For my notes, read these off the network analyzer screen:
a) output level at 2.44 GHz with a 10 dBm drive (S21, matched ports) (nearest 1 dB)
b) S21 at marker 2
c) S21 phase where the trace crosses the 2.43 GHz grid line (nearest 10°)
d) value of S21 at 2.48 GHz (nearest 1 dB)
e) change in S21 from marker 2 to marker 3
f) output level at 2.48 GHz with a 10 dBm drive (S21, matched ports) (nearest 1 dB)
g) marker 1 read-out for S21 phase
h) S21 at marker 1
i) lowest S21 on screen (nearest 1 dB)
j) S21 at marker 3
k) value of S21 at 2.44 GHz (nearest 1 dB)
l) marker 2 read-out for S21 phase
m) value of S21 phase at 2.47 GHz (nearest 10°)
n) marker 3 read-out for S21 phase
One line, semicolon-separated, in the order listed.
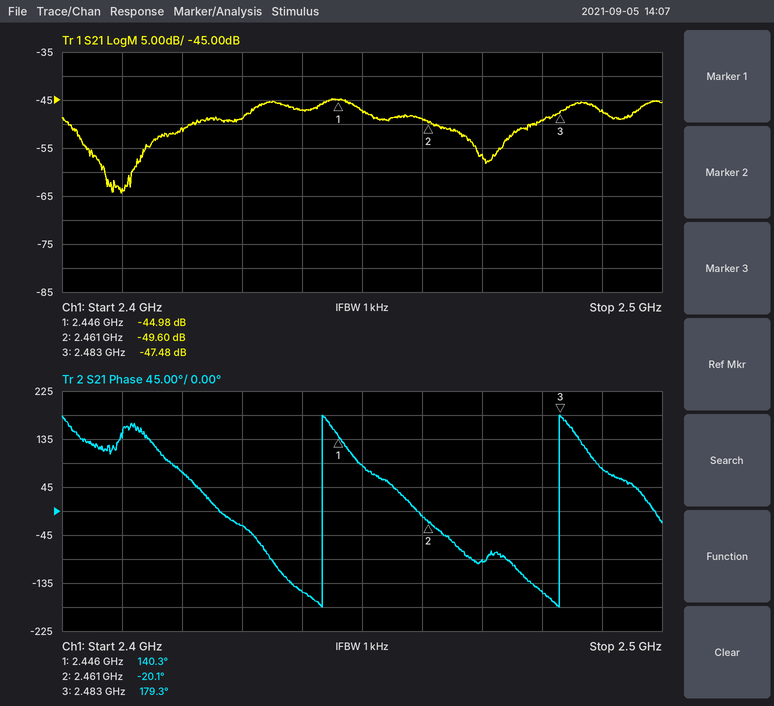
-37 dBm; -49.60 dB; -30°; -49 dB; 2.12 dB; -39 dBm; 140.3°; -44.98 dB; -64 dB; -47.48 dB; -47 dB; -20.1°; -90°; 179.3°
